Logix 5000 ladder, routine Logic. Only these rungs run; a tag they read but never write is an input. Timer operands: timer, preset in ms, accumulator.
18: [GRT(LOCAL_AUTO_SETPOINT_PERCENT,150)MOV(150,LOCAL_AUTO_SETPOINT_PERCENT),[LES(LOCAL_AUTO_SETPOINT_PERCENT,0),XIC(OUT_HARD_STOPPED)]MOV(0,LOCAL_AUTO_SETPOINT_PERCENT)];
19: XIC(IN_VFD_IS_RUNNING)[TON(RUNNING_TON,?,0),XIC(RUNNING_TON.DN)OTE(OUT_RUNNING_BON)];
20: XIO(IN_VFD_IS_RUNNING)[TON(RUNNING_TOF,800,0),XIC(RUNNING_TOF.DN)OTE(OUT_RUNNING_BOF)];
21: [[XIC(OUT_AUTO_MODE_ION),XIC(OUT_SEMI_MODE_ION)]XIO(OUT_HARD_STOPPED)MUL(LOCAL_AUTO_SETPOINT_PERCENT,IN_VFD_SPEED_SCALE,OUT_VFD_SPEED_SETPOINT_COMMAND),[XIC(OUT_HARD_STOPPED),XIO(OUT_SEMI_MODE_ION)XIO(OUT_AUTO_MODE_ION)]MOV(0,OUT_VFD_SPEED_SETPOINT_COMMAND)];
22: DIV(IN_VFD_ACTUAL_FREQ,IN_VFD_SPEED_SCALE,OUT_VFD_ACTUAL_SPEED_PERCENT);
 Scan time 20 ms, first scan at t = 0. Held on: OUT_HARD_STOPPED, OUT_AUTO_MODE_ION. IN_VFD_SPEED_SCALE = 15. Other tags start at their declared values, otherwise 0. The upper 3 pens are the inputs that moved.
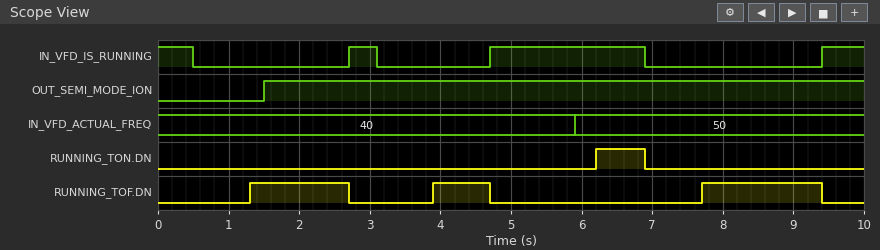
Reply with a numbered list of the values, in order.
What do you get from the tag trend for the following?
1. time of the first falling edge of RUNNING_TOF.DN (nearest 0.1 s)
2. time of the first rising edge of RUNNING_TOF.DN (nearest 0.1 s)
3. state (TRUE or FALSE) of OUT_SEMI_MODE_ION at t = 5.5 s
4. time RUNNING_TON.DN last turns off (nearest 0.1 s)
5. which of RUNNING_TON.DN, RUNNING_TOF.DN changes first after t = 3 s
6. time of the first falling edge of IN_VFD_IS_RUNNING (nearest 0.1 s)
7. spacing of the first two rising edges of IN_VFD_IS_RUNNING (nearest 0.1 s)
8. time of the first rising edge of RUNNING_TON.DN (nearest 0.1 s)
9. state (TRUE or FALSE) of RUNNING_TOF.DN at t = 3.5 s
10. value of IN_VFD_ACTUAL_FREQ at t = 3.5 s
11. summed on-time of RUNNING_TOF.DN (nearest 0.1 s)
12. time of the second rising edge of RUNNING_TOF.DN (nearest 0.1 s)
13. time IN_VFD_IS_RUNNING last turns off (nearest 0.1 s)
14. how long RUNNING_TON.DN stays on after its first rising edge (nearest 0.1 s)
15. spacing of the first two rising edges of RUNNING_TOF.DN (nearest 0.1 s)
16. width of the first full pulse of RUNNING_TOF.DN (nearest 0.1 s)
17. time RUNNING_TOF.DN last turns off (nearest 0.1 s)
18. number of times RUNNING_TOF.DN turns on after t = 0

1. 2.7 s
2. 1.3 s
3. TRUE
4. 6.9 s
5. RUNNING_TOF.DN
6. 0.5 s
7. 2.0 s
8. 6.2 s
9. FALSE
10. 40
11. 3.9 s
12. 3.9 s
13. 6.9 s
14. 0.7 s
15. 2.6 s
16. 1.4 s
17. 9.4 s
18. 3
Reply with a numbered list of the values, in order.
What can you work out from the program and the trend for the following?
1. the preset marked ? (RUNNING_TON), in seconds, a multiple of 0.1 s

1. 1.5 s
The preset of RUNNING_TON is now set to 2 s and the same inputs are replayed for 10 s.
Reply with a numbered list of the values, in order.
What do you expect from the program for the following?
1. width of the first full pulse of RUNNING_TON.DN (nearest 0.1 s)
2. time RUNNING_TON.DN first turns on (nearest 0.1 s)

1. 0.2 s
2. 6.7 s
